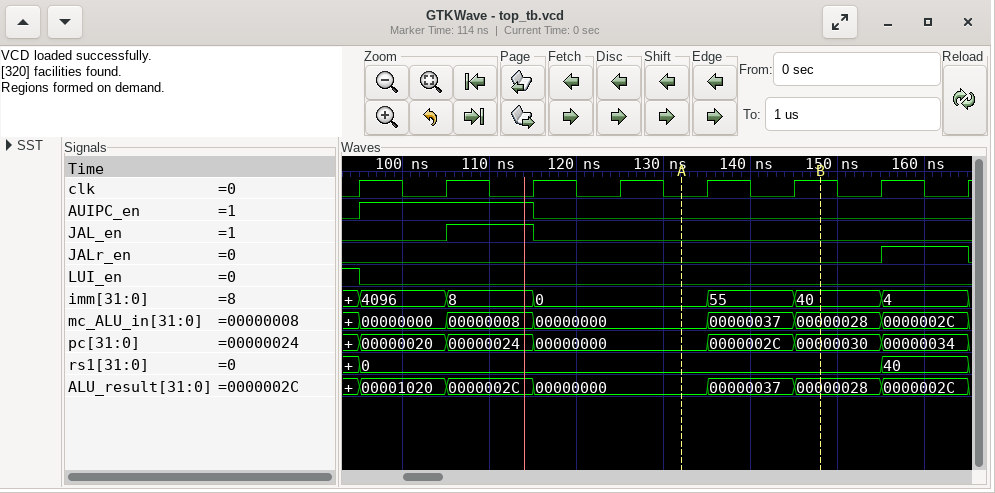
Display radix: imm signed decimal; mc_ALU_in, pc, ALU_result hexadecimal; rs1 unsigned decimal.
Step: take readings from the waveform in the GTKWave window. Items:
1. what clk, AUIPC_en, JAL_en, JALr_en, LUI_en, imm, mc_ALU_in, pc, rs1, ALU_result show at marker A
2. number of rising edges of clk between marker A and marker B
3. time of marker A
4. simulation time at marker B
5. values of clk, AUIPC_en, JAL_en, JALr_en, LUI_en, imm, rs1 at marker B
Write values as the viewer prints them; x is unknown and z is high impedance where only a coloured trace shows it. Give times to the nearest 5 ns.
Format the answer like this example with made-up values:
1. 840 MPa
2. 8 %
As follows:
1. clk=0, AUIPC_en=0, JAL_en=0, JALr_en=0, LUI_en=0, imm=0, mc_ALU_in=00000000, pc=00000000, rs1=0, ALU_result=00000000
2. 2
3. 130 ns
4. 150 ns
5. clk=1, AUIPC_en=0, JAL_en=0, JALr_en=0, LUI_en=0, imm=40, rs1=0
